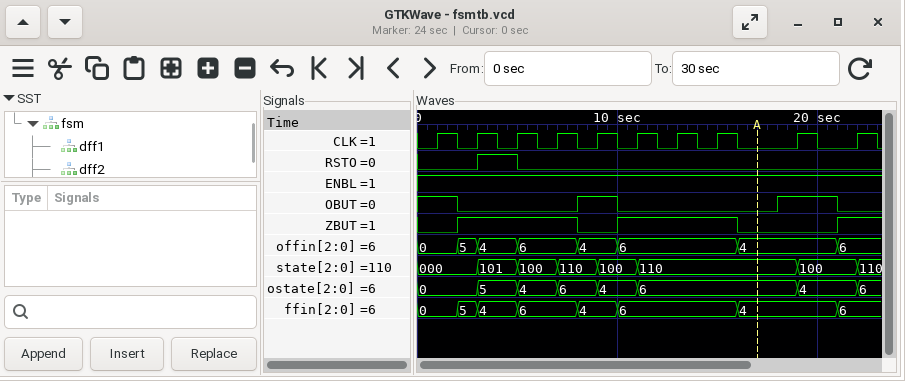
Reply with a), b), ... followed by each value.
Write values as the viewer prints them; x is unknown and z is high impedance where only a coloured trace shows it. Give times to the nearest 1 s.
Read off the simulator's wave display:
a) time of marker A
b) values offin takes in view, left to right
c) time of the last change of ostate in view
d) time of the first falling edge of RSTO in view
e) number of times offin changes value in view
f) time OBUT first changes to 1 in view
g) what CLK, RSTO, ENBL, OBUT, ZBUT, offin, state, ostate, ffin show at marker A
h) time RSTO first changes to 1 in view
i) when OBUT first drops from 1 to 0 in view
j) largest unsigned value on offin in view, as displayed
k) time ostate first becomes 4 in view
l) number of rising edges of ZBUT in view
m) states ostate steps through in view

a) 17 s
b) 0, 5, 4, 6, 4, 6, 4, 6
c) 22 s
d) 5 s
e) 7
f) 8 s
g) CLK=0, RSTO=0, ENBL=1, OBUT=0, ZBUT=0, offin=4, state=110, ostate=6, ffin=4
h) 3 s
i) 2 s
j) 6
k) 5 s
l) 3
m) 0, 5, 4, 6, 4, 6, 4, 6
